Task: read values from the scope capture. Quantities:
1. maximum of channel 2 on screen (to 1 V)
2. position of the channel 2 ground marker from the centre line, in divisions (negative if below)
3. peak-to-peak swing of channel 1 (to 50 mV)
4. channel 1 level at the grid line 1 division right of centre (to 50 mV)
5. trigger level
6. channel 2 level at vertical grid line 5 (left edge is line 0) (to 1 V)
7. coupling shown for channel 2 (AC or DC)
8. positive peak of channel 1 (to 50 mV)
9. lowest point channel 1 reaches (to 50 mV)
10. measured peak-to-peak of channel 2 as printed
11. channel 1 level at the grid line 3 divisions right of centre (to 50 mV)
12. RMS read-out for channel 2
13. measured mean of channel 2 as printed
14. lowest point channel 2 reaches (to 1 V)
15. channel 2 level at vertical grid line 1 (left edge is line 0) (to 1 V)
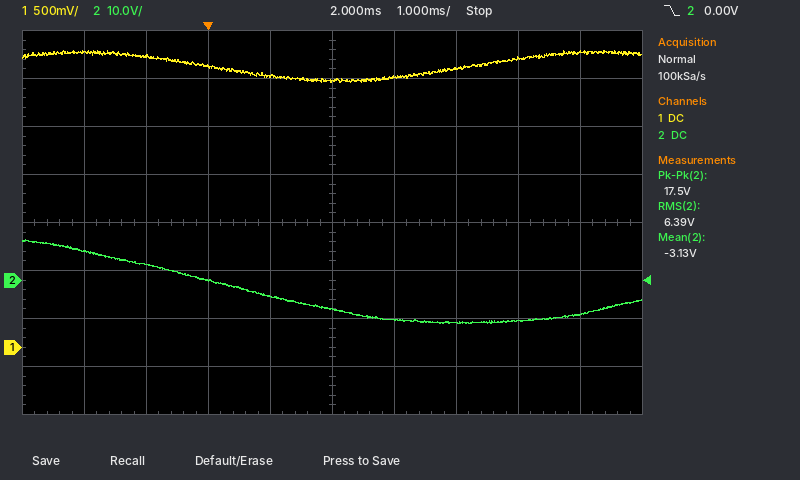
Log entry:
8 V
-1.2 div
350 mV
2.80 V
0.00 V
-6 V
DC
3.10 V
2.75 V
17.5 V
3.00 V
6.39 V
-3.13 V
-9 V
6 V
